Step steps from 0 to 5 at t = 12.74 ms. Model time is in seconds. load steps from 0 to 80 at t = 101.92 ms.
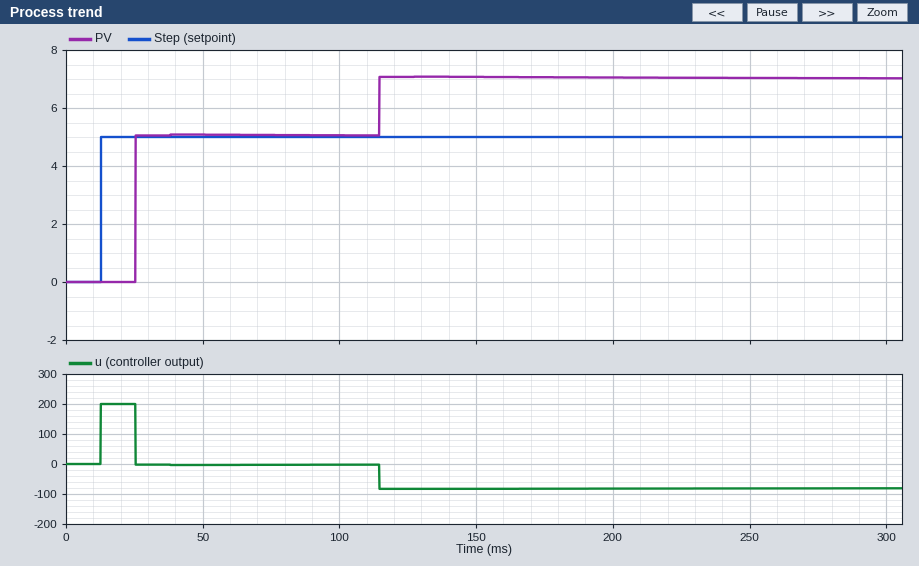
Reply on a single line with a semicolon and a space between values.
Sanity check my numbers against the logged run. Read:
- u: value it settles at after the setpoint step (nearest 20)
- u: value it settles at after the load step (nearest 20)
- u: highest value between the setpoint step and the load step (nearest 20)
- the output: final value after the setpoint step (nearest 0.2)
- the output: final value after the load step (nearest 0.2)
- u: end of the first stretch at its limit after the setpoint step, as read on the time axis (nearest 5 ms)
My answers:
0; -80; 200; 5.0; 7.0; 25 ms
